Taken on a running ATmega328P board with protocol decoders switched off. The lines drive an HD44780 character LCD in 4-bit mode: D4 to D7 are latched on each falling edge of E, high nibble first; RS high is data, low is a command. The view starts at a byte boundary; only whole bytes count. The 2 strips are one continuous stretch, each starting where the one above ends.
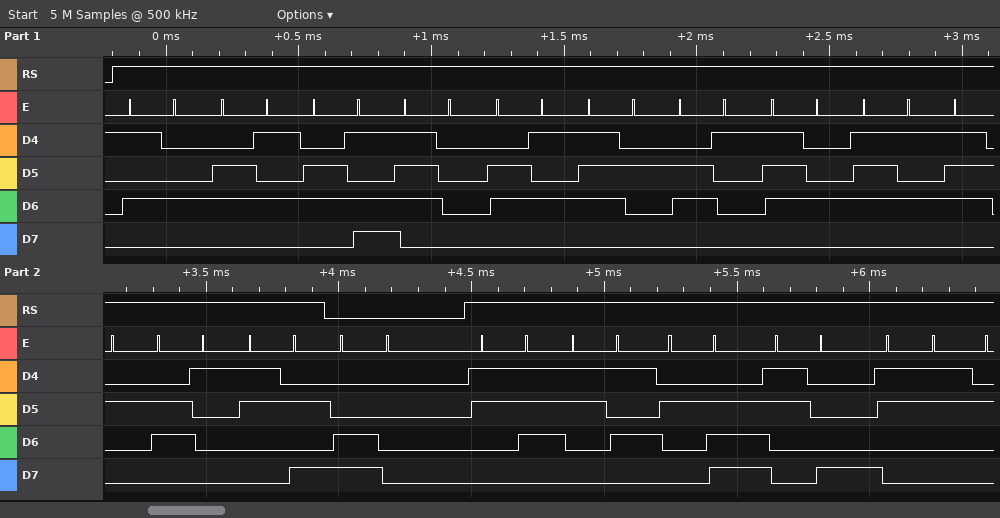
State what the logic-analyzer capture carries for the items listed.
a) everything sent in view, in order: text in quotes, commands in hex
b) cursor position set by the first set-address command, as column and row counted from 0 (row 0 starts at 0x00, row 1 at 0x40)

"Temperatura:" 0xC0 "75.83"
column 0, row 1
